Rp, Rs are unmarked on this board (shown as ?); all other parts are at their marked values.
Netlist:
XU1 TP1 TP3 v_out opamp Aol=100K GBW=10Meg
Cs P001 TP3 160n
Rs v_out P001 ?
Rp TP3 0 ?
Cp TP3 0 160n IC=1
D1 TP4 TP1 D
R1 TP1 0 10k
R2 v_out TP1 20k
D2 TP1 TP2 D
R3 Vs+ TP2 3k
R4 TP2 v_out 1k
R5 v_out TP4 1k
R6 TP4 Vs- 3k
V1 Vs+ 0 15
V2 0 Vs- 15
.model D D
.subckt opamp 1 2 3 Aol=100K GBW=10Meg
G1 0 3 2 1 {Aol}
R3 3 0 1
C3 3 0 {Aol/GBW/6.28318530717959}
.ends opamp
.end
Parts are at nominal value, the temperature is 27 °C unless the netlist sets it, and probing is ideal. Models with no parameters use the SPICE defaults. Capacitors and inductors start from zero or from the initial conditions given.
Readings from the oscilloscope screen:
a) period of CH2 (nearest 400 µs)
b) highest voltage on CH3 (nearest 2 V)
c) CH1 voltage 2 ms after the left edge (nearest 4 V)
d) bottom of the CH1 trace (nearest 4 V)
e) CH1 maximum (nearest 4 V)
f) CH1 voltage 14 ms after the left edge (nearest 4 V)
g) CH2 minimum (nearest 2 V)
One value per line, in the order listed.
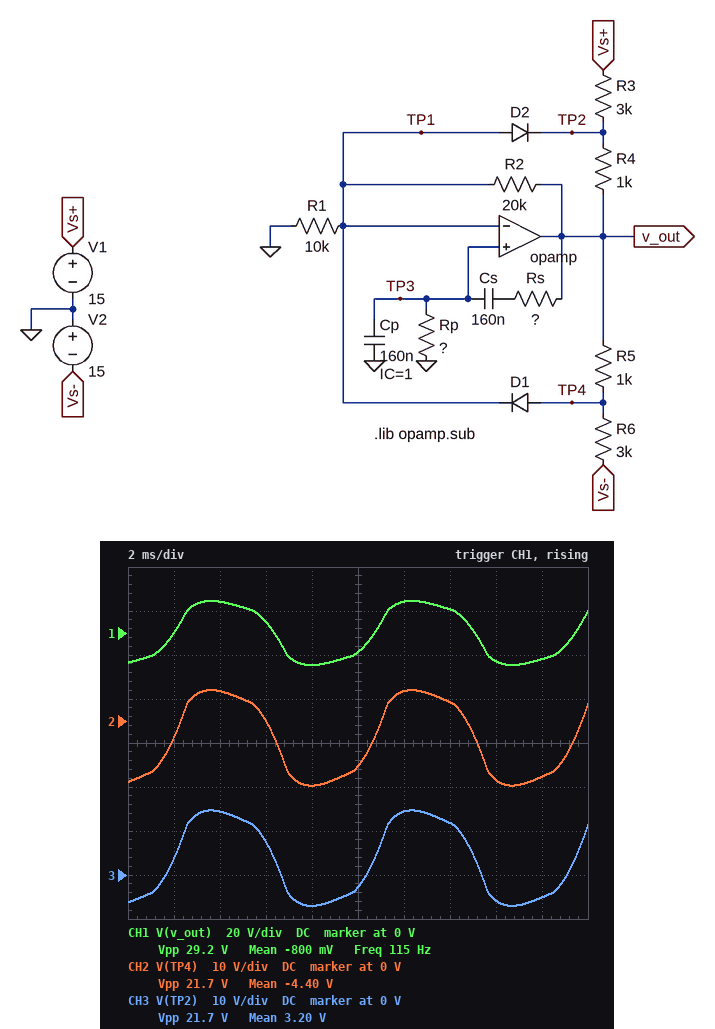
8.8 ms
14 V
0 V
-16 V
16 V
12 V
-14 V
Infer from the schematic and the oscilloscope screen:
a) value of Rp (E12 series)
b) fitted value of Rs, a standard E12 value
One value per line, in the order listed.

12 kΩ
5.6 kΩ
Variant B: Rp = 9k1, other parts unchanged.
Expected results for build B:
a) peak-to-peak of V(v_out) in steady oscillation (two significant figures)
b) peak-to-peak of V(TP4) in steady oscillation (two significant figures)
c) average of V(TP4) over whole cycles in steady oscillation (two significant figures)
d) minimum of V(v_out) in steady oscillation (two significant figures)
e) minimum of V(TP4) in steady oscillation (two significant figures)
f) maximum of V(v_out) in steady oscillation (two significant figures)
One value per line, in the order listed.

26 V
20 V
-3.8 V
-13 V
-14 V
13 V
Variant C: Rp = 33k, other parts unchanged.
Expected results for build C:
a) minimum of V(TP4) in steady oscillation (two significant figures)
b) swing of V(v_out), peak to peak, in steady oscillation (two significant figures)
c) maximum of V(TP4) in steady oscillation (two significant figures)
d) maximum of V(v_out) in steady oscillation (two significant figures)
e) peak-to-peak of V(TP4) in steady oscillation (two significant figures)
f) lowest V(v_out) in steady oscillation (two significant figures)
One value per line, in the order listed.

-18 V
38 V
10 V
19 V
28 V
-19 V
